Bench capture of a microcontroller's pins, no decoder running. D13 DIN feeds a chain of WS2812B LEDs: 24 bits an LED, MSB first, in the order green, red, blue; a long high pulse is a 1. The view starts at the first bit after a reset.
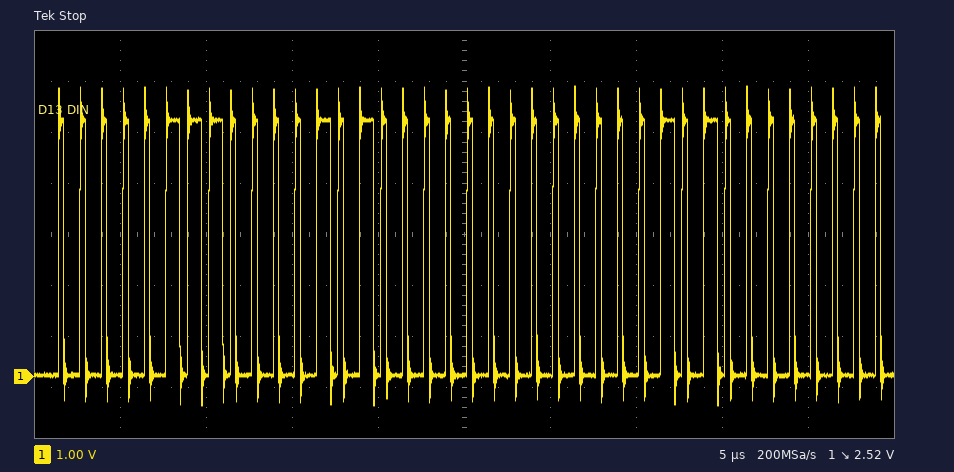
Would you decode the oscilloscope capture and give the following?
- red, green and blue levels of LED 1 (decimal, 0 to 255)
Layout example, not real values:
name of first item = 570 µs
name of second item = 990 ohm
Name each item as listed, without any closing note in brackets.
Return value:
red, green and blue levels of LED 1 = 10, 7, 0
